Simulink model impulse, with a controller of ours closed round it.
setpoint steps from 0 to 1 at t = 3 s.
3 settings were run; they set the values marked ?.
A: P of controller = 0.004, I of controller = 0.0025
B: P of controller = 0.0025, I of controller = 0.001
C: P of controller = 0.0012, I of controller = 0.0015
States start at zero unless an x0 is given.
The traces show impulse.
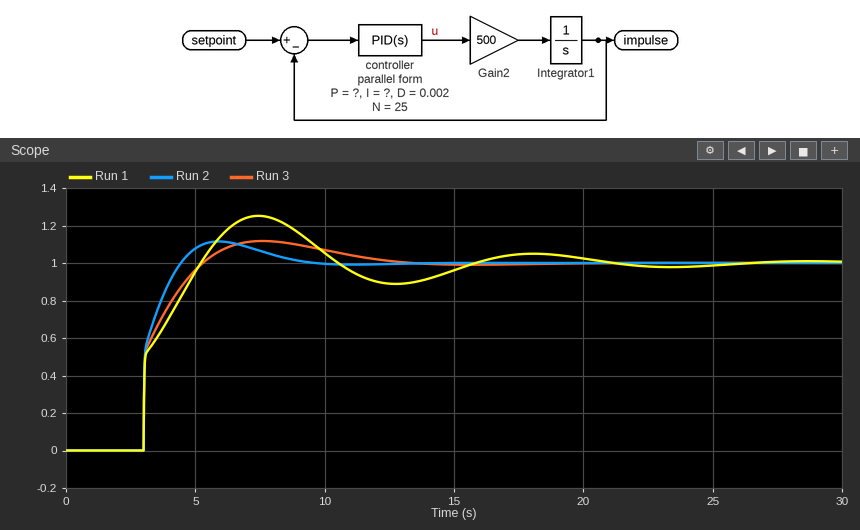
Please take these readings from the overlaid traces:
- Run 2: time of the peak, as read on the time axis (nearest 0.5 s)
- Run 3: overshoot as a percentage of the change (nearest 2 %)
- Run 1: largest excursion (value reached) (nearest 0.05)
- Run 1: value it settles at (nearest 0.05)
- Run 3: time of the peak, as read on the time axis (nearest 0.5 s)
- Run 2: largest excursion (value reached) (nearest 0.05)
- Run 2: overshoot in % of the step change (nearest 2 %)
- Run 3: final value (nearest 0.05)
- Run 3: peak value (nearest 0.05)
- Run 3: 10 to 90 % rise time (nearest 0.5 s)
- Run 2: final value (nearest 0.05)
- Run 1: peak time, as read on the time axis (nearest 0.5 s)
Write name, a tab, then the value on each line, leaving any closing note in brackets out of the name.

Run 2: time of the peak, as read on the time axis	6.0 s
Run 3: overshoot as a percentage of the change	12 %
Run 1: largest excursion (value reached)	1.25
Run 1: value it settles at	1.00
Run 3: time of the peak, as read on the time axis	7.5 s
Run 2: largest excursion (value reached)	1.10
Run 2: overshoot in % of the step change	12 %
Run 3: final value	1.00
Run 3: peak value	1.10
Run 3: 10 to 90 % rise time	1.5 s
Run 2: final value	1.00
Run 1: peak time, as read on the time axis	7.5 s
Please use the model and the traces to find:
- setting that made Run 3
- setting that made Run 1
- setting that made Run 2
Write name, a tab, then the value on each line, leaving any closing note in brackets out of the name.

setting that made Run 3	B
setting that made Run 1	C
setting that made Run 2	A
